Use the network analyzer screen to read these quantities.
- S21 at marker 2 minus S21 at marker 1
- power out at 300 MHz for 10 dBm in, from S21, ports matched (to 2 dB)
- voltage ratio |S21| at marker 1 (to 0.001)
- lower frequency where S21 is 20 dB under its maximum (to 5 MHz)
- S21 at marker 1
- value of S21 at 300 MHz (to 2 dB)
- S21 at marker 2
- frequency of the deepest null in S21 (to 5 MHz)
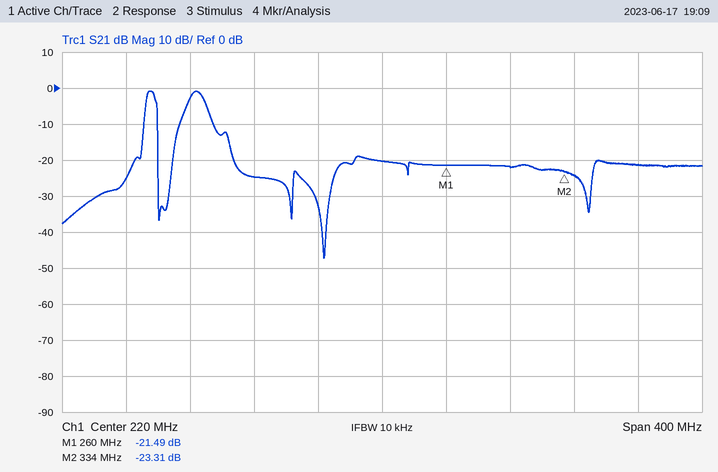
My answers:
-1.82 dB
-12 dBm
0.084
65 MHz
-21.49 dB
-22 dB
-23.31 dB
185 MHz
